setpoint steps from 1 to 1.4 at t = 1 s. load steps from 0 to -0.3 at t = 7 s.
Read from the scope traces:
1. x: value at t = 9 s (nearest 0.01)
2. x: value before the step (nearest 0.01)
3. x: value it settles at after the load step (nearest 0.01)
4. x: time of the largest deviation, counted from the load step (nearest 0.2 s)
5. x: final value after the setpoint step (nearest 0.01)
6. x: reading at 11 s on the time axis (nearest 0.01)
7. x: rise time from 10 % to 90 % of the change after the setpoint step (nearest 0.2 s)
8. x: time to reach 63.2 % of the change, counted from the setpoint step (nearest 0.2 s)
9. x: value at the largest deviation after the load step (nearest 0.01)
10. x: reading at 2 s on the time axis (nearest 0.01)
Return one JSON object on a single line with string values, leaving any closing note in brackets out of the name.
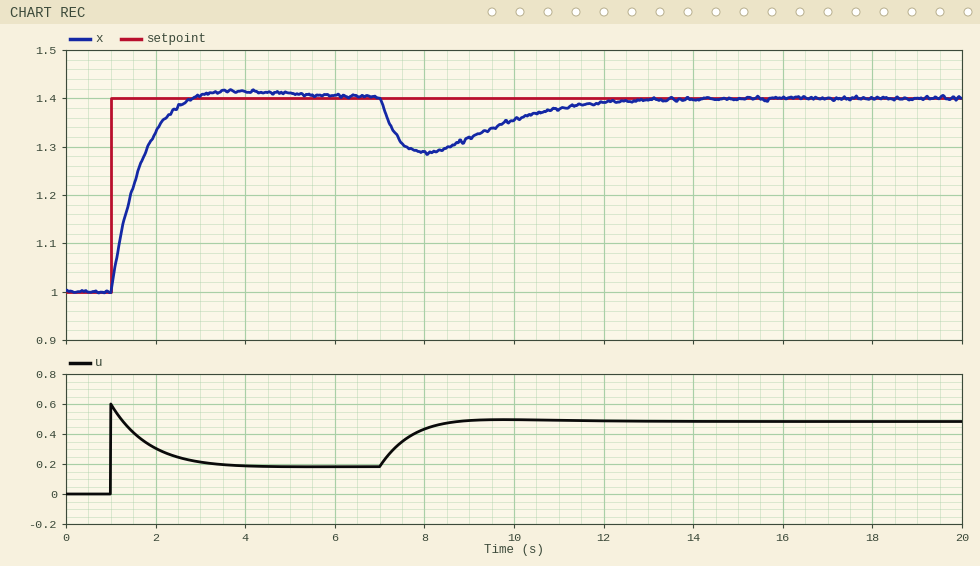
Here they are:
{"x: value at t = 9 s": "1.32", "x: value before the step": "1.00", "x: value it settles at after the load step": "1.40", "x: time of the largest deviation, counted from the load step": "1.0 s", "x: final value after the setpoint step": "1.40", "x: reading at 11 s on the time axis": "1.38", "x: rise time from 10 % to 90 % of the change after the setpoint step": "1.2 s", "x: time to reach 63.2 % of the change, counted from the setpoint step": "0.6 s", "x: value at the largest deviation after the load step": "1.29", "x: reading at 2 s on the time axis": "1.33"}
